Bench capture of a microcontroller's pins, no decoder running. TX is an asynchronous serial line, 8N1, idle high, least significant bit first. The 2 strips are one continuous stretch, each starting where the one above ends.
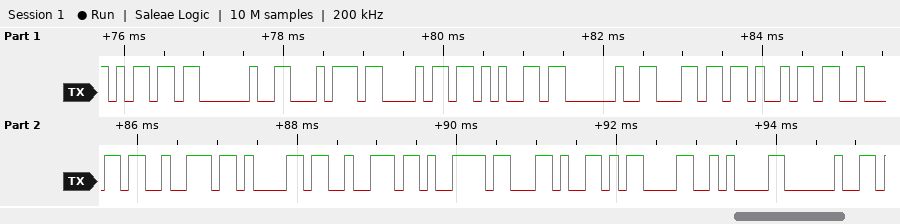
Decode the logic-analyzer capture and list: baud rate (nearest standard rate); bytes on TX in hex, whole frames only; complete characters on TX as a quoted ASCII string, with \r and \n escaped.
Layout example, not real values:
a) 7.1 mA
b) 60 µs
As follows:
a) 9600 baud
b) 6D 20 74 68 65 20 6C 69 62 72 61 72 79 2C 0D 0A 20
c) "m the library,\r\n "
